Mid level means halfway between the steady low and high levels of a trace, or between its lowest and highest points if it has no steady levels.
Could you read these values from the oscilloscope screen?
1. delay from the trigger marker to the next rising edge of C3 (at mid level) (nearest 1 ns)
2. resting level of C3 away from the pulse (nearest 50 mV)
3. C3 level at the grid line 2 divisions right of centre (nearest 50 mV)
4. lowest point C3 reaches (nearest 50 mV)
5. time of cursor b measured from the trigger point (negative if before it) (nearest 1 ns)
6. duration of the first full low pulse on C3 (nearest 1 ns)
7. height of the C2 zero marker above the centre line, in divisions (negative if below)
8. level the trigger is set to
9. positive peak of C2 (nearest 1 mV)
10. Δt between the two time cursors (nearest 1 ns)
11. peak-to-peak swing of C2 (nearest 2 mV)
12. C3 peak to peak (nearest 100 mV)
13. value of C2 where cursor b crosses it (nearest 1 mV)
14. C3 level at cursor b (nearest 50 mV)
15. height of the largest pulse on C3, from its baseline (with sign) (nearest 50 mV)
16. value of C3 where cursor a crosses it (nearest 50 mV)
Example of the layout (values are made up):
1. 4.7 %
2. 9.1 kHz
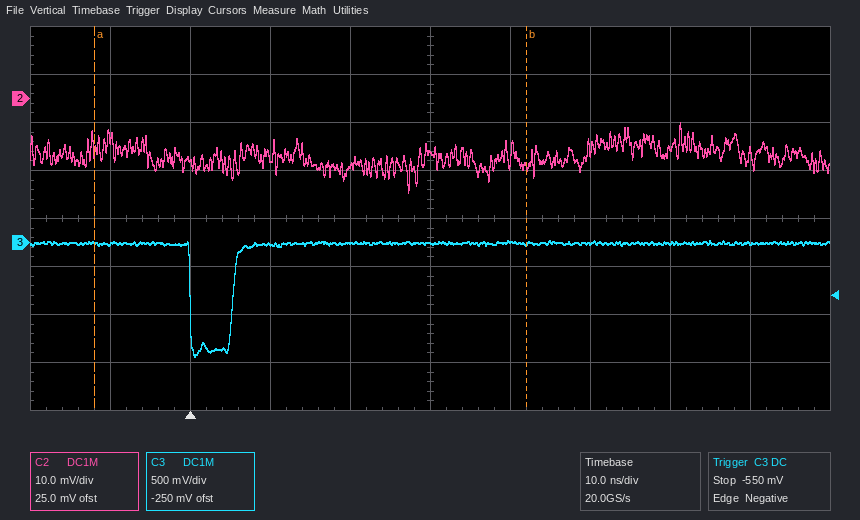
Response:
1. 5 ns
2. 0 mV
3. 0 mV
4. -1.20 V
5. +42 ns
6. 5 ns
7. +2.5 div
8. -550 mV
9. -5 mV
10. 54 ns
11. 14 mV
12. 1.20 V
13. -14 mV
14. 0 mV
15. -1.20 V
16. 0 mV
